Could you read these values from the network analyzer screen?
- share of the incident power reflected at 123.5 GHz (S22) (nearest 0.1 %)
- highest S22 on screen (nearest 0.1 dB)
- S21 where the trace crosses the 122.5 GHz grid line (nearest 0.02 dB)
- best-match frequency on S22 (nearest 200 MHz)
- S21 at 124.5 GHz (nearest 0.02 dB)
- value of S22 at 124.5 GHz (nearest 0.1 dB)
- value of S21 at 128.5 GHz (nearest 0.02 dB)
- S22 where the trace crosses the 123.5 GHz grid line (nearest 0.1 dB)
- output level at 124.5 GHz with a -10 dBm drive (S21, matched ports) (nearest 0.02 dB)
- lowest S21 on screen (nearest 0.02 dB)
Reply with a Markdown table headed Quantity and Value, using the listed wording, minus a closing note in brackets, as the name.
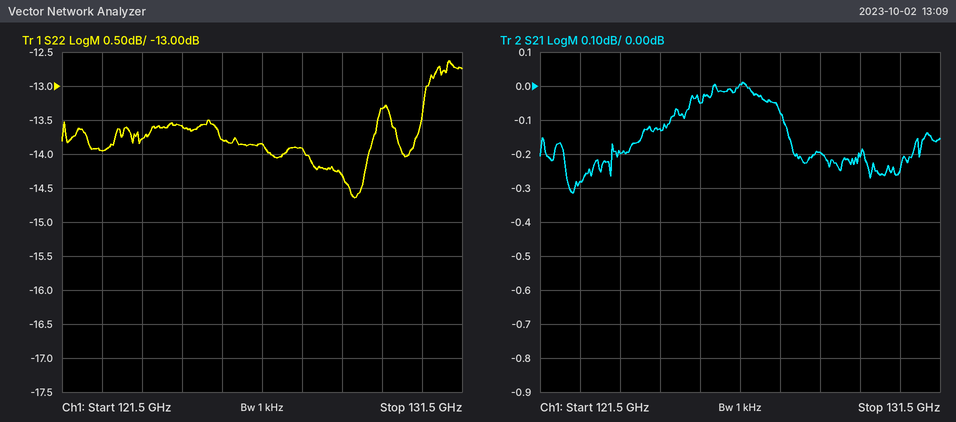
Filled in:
| Quantity | Value |
|---|---|
| share of the incident power reflected at 123.5 GHz (S22) | 4.2 % |
| highest S22 on screen | -12.6 dB |
| S21 where the trace crosses the 122.5 GHz grid line | -0.28 dB |
| best-match frequency on S22 | 128.8 GHz |
| S21 at 124.5 GHz | -0.12 dB |
| value of S22 at 124.5 GHz | -13.6 dB |
| value of S21 at 128.5 GHz | -0.20 dB |
| S22 where the trace crosses the 123.5 GHz grid line | -13.8 dB |
| output level at 124.5 GHz with a -10 dBm drive (S21, matched ports) | -10.12 dBm |
| lowest S21 on screen | -0.32 dB |
